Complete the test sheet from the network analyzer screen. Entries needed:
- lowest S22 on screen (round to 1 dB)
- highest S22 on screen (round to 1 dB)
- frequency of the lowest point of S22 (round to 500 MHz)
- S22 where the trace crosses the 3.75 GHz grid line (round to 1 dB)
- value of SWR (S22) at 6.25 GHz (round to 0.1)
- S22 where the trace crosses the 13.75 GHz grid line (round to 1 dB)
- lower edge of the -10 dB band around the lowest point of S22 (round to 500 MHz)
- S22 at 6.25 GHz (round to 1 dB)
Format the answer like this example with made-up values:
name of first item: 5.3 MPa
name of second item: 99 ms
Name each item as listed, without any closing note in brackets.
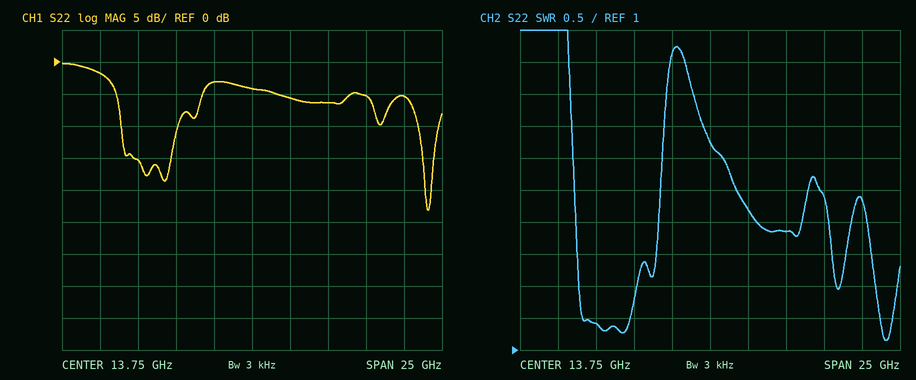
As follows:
lowest S22 on screen: -23 dB
highest S22 on screen: 0 dB
frequency of the lowest point of S22: 25.5 GHz
S22 where the trace crosses the 3.75 GHz grid line: -2 dB
value of SWR (S22) at 6.25 GHz: 1.4
S22 where the trace crosses the 13.75 GHz grid line: -4 dB
lower edge of the -10 dB band around the lowest point of S22: 24.5 GHz
S22 at 6.25 GHz: -15 dB
